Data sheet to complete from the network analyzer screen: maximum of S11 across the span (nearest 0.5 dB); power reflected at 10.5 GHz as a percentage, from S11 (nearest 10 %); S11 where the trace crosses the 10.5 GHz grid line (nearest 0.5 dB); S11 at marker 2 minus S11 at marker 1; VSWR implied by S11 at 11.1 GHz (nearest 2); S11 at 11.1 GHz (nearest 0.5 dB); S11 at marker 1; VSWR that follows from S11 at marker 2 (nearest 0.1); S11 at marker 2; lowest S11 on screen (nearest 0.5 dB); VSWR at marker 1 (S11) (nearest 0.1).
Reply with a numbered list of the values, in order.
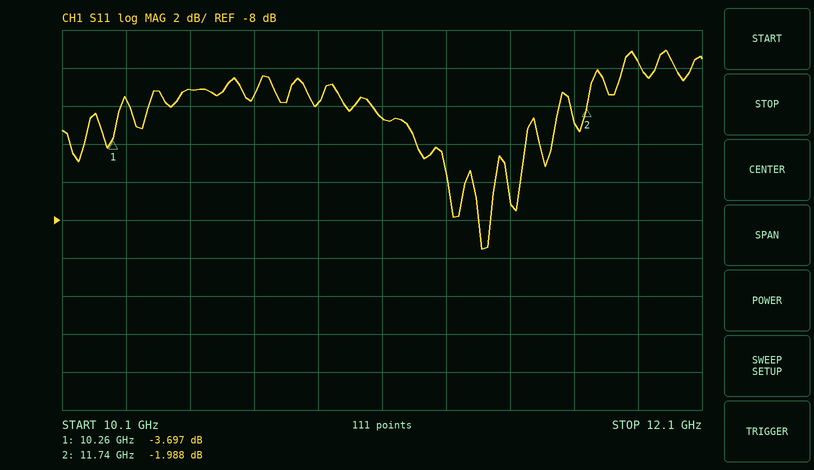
1. 1.0 dB
2. 80 %
3. -1.0 dB
4. 1.709 dB
5. 6
6. -2.5 dB
7. -3.697 dB
8. 8.8
9. -1.988 dB
10. -9.5 dB
11. 4.8
